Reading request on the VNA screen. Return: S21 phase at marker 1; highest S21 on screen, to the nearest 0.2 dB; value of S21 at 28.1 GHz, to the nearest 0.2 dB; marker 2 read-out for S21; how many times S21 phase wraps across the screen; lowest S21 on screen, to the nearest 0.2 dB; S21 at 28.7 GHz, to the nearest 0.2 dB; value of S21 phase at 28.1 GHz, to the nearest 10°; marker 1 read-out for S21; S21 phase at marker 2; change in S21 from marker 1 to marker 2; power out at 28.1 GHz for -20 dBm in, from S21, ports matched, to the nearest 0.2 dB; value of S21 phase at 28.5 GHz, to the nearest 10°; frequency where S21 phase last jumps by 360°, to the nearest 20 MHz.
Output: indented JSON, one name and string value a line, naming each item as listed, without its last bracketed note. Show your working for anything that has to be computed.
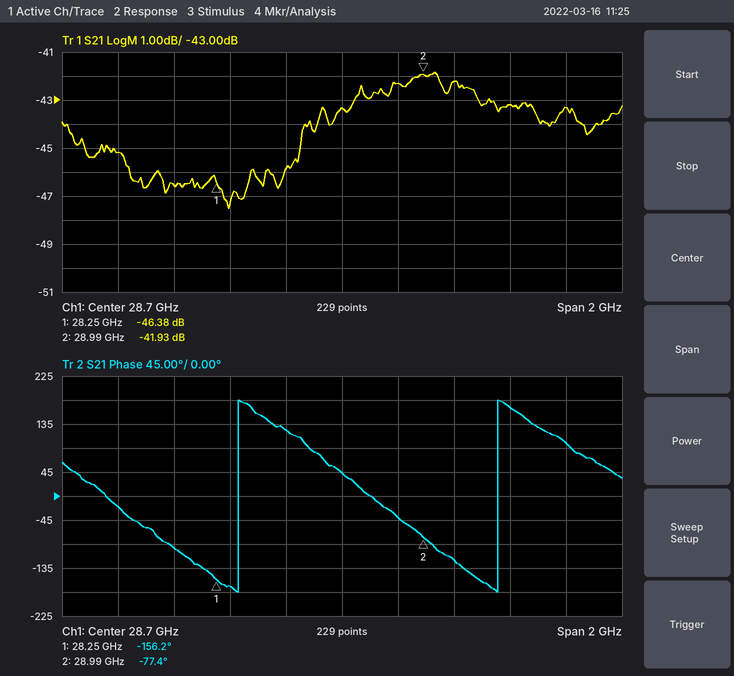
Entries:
{
  "S21 phase at marker 1": "-156.2°",
  "highest S21 on screen, to the nearest 0.2 dB": "-41.8 dB",
  "value of S21 at 28.1 GHz, to the nearest 0.2 dB": "-46.6 dB",
  "marker 2 read-out for S21": "-41.93 dB",
  "how many times S21 phase wraps across the screen": "2",
  "lowest S21 on screen, to the nearest 0.2 dB": "-47.6 dB",
  "S21 at 28.7 GHz, to the nearest 0.2 dB": "-43.4 dB",
  "value of S21 phase at 28.1 GHz, to the nearest 10°": "-100°",
  "marker 1 read-out for S21": "-46.38 dB",
  "S21 phase at marker 2": "-77.4°",
  "change in S21 from marker 1 to marker 2": "-41.93 − (-46.38) = 4.45 dB",
  "power out at 28.1 GHz for -20 dBm in, from S21, ports matched, to the nearest 0.2 dB": "-20 dBm + (-46.6 dB) = -66.6 dBm",
  "value of S21 phase at 28.5 GHz, to the nearest 10°": "120°",
  "frequency where S21 phase last jumps by 360°, to the nearest 20 MHz": "29.26 GHz"
}
